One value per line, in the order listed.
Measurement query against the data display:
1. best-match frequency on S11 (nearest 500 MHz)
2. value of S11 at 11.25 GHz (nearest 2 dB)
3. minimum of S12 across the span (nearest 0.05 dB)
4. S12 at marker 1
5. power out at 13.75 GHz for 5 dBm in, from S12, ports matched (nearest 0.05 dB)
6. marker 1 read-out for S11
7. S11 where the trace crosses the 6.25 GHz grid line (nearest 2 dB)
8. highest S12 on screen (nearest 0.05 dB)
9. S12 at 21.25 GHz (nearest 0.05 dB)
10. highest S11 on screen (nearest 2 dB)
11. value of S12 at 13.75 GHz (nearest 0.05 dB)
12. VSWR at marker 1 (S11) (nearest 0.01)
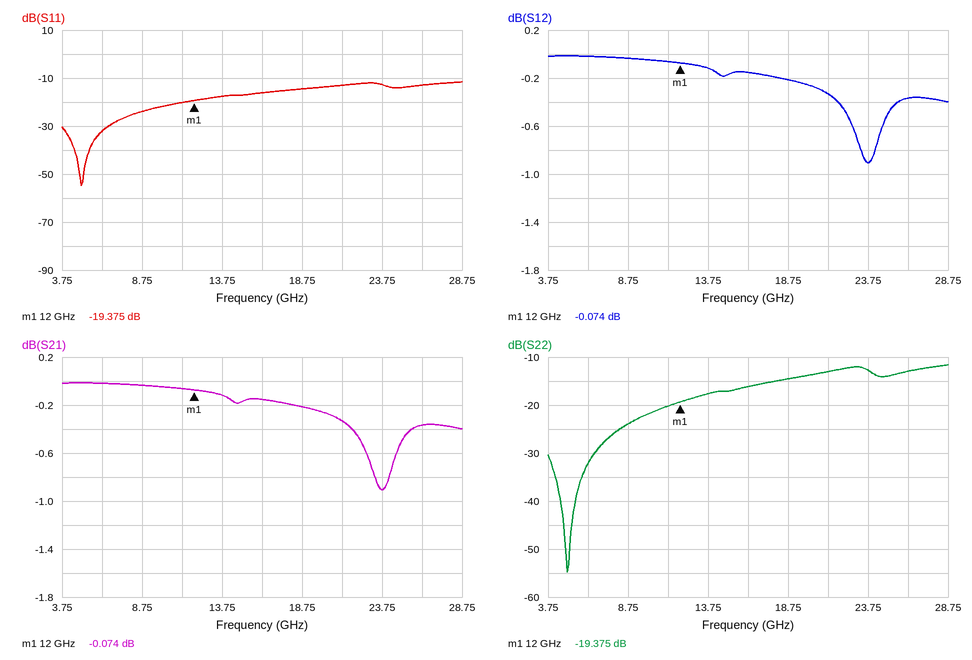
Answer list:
5.0 GHz
-20 dB
-0.90 dB
-0.074 dB
4.90 dBm
-19.375 dB
-32 dB
0.00 dB
-0.35 dB
-12 dB
-0.10 dB
1.24
